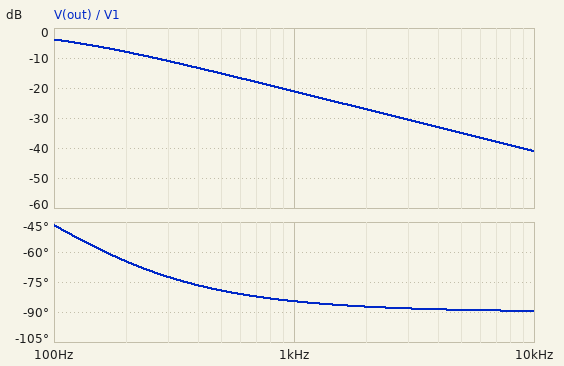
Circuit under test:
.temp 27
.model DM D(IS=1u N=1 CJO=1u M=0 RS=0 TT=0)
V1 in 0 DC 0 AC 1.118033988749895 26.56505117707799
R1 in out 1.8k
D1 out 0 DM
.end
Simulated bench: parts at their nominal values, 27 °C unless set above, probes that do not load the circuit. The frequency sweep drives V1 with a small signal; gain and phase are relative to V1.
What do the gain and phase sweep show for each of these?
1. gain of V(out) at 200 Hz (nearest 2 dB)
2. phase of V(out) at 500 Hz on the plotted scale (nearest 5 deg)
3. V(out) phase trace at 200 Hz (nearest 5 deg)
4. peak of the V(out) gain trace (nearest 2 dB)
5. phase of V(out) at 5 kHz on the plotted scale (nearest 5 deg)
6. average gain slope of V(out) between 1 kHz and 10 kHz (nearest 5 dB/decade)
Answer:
-8 dB
-80 deg
-65 deg
-4 dB
-90 deg
-20 dB/decade
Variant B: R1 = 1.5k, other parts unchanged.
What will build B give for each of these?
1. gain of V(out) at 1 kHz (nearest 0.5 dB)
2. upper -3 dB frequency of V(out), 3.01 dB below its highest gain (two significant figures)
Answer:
-19.5 dB
110 Hz
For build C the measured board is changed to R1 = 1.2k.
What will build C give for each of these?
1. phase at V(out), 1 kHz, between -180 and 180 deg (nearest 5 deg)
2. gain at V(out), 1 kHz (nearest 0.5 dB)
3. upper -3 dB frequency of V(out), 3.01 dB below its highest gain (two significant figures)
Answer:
-80 deg
-17.5 dB
140 Hz
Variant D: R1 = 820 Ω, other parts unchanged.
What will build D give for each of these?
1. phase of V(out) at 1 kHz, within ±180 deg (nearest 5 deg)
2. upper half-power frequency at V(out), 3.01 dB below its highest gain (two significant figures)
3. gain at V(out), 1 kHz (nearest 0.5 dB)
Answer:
-80 deg
200 Hz
-14.5 dB
